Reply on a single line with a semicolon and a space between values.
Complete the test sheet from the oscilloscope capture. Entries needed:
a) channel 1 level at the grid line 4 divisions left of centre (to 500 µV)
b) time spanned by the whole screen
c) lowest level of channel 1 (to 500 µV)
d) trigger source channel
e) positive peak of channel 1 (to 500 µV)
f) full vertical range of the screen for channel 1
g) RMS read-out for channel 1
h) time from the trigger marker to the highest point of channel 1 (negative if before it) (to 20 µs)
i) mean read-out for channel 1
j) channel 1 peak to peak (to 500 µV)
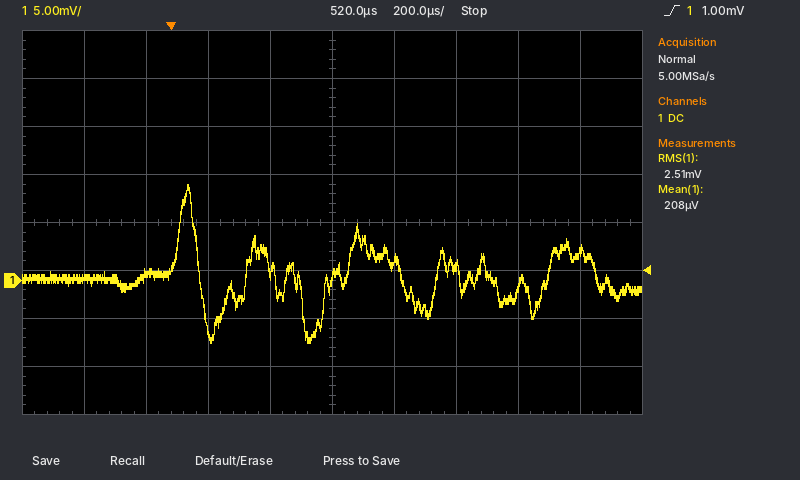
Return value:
0.0 mV; 2 ms; -6.5 mV; channel 1; 10.0 mV; 40 mV; 2.51 mV; +60 µs; 208 µV; 16.5 mV
